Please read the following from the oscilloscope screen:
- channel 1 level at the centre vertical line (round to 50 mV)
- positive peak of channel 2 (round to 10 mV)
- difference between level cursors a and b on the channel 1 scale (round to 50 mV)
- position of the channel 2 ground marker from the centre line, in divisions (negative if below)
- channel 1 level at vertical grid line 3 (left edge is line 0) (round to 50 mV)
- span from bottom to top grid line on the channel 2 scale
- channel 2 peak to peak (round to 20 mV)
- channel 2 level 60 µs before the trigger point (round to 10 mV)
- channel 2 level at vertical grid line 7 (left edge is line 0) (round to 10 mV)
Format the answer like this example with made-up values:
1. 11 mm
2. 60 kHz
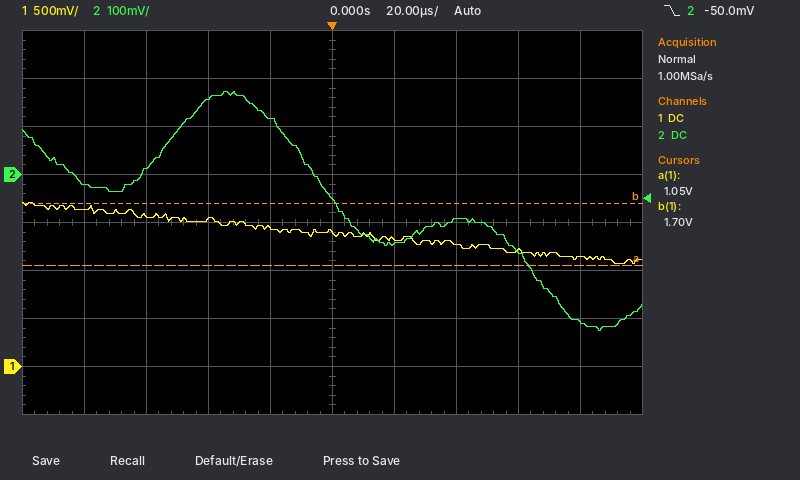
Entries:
1. 1.40 V
2. 170 mV
3. 650 mV
4. +1.0 div
5. 1.55 V
6. 800 mV
7. 500 mV
8. 10 mV
9. -90 mV
